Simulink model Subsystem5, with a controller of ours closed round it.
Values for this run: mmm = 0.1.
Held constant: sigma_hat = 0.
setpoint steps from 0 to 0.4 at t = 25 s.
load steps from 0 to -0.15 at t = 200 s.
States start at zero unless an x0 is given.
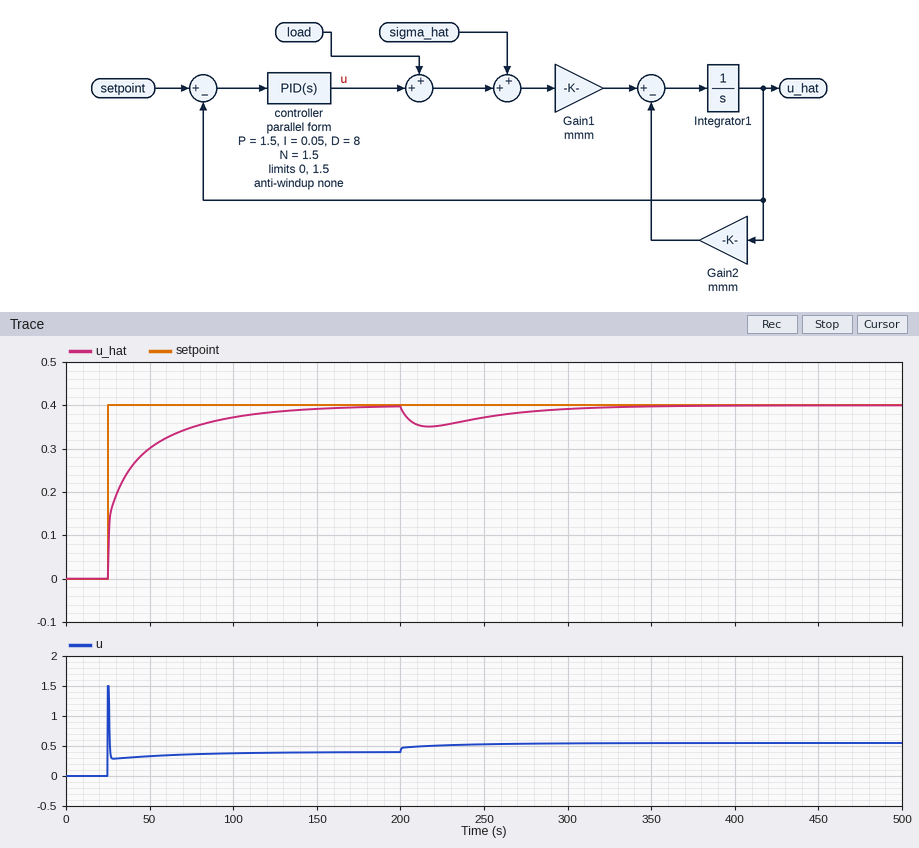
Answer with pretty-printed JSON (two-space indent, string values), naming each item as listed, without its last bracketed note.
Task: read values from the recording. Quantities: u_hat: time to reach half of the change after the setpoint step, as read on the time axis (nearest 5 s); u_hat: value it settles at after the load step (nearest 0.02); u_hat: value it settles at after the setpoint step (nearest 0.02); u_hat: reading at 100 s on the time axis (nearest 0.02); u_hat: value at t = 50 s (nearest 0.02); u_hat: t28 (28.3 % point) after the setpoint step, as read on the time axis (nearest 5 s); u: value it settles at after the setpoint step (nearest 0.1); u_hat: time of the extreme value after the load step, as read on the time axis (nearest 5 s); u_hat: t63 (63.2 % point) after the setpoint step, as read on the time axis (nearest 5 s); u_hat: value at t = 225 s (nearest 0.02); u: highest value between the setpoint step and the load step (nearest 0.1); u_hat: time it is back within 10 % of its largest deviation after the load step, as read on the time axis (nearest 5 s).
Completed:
{
  "u_hat: time to reach half of the change after the setpoint step, as read on the time axis": "30 s",
  "u_hat: value it settles at after the load step": "0.40",
  "u_hat: value it settles at after the setpoint step": "0.40",
  "u_hat: reading at 100 s on the time axis": "0.38",
  "u_hat: value at t = 50 s": "0.30",
  "u_hat: t28 (28.3 % point) after the setpoint step, as read on the time axis": "25 s",
  "u: value it settles at after the setpoint step": "0.4",
  "u_hat: time of the extreme value after the load step, as read on the time axis": "215 s",
  "u_hat: t63 (63.2 % point) after the setpoint step, as read on the time axis": "40 s",
  "u_hat: value at t = 225 s": "0.36",
  "u: highest value between the setpoint step and the load step": "1.5",
  "u_hat: time it is back within 10 % of its largest deviation after the load step, as read on the time axis": "325 s"
}
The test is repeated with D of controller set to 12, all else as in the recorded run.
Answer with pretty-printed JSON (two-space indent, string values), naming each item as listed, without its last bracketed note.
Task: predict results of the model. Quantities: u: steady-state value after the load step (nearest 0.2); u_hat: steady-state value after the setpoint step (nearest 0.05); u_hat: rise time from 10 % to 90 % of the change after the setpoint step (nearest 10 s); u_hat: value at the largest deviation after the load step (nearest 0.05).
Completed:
{
  "u: steady-state value after the load step": "0.6",
  "u_hat: steady-state value after the setpoint step": "0.40",
  "u_hat: rise time from 10 % to 90 % of the change after the setpoint step": "60 s",
  "u_hat: value at the largest deviation after the load step": "0.35"
}
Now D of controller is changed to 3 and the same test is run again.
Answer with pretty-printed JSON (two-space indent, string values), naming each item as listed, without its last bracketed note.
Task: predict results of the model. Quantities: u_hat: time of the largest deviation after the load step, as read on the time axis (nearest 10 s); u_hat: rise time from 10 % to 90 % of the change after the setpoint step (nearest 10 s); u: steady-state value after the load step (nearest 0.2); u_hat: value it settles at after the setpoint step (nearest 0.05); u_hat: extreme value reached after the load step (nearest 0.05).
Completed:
{
  "u_hat: time of the largest deviation after the load step, as read on the time axis": "210 s",
  "u_hat: rise time from 10 % to 90 % of the change after the setpoint step": "60 s",
  "u: steady-state value after the load step": "0.6",
  "u_hat: value it settles at after the setpoint step": "0.40",
  "u_hat: extreme value reached after the load step": "0.35"
}
